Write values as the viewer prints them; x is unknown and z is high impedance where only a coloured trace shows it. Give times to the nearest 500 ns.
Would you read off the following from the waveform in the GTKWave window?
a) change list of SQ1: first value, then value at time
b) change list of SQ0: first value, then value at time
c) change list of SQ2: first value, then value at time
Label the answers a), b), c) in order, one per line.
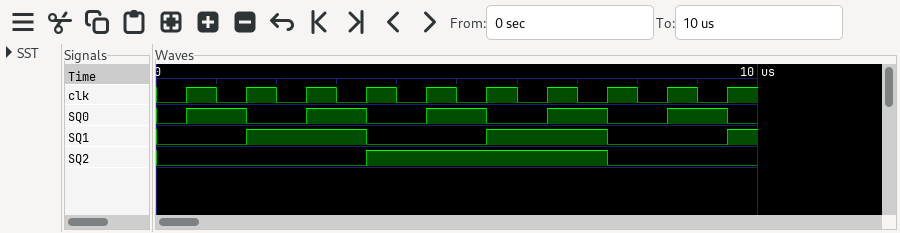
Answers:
a) 0, 1 at 1500 ns, 0 at 3500 ns, 1 at 5500 ns, 0 at 7500 ns, 1 at 9500 ns
b) 0, 1 at 500 ns, 0 at 1500 ns, 1 at 2500 ns, 0 at 3500 ns, 1 at 4500 ns, 0 at 5500 ns, 1 at 6500 ns, 0 at 7500 ns, 1 at 8500 ns, 0 at 9500 ns
c) 0, 1 at 3500 ns, 0 at 7500 ns
